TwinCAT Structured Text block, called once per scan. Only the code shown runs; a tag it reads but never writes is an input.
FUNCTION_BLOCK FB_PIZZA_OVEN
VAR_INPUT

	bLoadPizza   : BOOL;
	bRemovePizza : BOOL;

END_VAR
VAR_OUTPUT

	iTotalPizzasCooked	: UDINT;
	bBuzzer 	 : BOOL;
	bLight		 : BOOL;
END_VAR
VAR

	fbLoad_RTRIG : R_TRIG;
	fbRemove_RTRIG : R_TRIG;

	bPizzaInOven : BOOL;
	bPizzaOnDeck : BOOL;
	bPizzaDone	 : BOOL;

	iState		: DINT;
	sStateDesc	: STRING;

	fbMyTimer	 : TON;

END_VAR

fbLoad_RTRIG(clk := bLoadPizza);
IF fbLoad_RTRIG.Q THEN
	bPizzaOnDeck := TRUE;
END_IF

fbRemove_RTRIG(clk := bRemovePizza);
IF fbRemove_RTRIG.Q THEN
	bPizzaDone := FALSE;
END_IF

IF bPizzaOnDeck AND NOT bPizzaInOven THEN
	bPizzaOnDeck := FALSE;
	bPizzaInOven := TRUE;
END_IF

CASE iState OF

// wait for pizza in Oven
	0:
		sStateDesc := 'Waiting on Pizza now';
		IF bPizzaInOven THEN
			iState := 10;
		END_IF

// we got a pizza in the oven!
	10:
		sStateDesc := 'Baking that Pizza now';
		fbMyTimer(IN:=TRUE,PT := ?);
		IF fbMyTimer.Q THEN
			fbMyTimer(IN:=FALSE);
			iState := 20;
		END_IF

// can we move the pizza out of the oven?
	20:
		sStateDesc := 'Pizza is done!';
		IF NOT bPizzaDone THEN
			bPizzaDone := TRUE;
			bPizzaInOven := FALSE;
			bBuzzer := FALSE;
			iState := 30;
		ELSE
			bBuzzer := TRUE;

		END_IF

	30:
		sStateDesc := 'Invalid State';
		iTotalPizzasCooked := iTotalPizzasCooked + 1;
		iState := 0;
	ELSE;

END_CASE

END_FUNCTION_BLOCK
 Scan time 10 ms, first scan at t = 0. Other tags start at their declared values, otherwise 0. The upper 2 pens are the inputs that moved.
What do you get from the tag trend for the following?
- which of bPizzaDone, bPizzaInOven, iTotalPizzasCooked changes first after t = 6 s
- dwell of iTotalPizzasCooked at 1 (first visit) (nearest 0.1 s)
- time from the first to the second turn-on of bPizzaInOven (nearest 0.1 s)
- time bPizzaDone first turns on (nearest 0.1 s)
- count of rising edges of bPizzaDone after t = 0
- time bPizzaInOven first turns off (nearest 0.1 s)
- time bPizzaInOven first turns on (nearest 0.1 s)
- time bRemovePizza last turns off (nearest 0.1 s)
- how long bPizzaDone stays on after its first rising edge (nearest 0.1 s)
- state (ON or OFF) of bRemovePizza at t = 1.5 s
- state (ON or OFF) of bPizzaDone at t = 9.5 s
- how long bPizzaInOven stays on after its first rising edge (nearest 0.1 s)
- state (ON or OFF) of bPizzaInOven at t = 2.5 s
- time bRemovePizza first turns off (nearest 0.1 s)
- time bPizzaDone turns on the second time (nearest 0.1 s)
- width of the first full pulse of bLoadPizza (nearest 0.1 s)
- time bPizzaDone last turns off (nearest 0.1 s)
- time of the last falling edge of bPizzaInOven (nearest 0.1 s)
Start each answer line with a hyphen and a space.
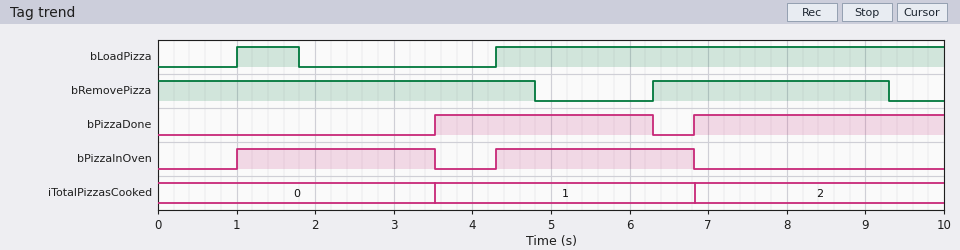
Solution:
- bPizzaDone
- 3.3 s
- 3.3 s
- 3.5 s
- 2
- 3.5 s
- 1.0 s
- 9.3 s
- 2.8 s
- ON
- ON
- 2.5 s
- ON
- 4.8 s
- 6.8 s
- 0.8 s
- 6.3 s
- 6.8 s
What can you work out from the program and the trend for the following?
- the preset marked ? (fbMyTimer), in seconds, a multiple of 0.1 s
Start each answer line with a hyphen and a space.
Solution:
- 2.5 s
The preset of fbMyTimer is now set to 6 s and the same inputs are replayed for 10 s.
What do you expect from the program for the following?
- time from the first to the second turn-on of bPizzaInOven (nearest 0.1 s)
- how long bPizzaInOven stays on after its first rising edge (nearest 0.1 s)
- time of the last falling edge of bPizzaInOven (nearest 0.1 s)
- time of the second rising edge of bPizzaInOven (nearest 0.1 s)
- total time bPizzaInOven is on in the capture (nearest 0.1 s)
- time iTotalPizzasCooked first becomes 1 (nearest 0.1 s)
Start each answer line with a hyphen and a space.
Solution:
- 6.0 s
- 6.0 s
- 7.0 s
- 7.0 s
- 9.0 s
- 7.0 s
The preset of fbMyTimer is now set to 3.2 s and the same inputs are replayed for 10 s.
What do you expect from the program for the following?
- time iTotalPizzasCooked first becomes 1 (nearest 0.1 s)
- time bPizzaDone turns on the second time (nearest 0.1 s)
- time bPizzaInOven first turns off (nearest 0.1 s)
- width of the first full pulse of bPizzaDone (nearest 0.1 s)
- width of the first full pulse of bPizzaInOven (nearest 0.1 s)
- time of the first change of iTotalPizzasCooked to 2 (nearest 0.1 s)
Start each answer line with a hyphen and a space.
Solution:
- 4.2 s
- 7.5 s
- 4.2 s
- 2.1 s
- 3.2 s
- 7.5 s
